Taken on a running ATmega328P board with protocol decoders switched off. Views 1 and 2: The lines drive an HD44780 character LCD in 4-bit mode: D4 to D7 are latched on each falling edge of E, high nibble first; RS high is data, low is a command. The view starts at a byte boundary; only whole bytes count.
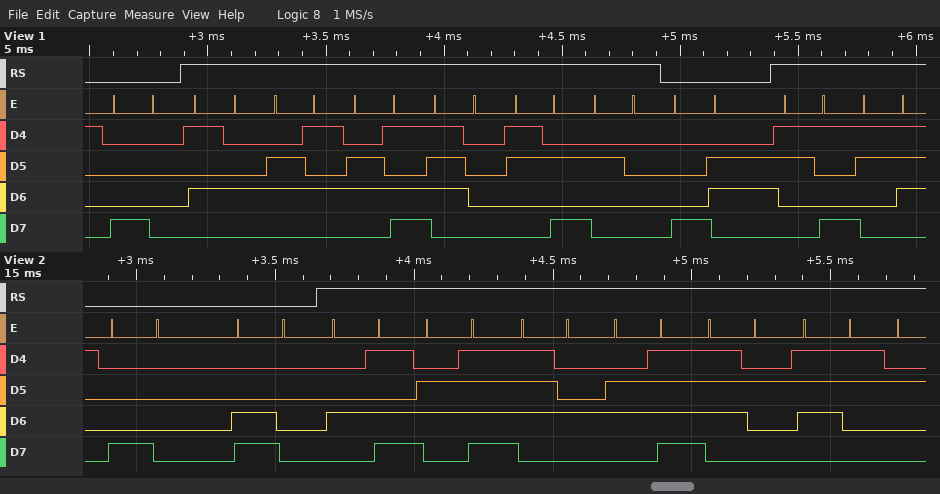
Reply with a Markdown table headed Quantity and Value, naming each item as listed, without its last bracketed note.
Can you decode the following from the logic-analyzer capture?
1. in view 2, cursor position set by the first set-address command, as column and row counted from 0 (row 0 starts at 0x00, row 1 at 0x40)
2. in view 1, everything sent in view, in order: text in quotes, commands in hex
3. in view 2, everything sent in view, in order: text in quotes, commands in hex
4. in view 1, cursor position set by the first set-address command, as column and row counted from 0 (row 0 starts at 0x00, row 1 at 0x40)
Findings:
| Quantity | Value |
|---|---|
| in view 2, cursor position set by the first set-address command, as column and row counted from 0 | column 0, row 0 |
| in view 1, everything sent in view, in order: text in quotes, commands in hex | 0x80 "Temp: " 0x86 "97" |
| in view 2, everything sent in view, in order: text in quotes, commands in hex | 0x80 0xC0 "Motors" |
| in view 1, cursor position set by the first set-address command, as column and row counted from 0 | column 0, row 0 |
